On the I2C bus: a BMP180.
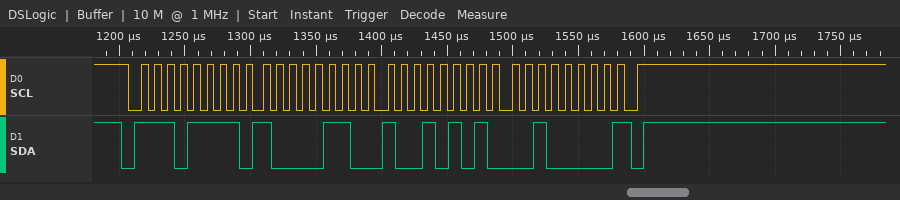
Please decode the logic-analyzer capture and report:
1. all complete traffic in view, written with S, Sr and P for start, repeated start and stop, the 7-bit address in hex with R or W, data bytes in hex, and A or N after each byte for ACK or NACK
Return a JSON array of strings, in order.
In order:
["S 77R A 86 A 95 A 20 N P"]
